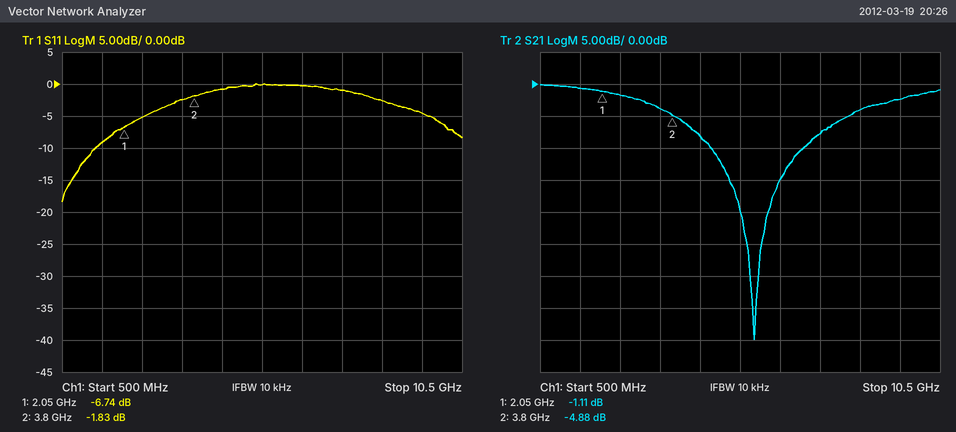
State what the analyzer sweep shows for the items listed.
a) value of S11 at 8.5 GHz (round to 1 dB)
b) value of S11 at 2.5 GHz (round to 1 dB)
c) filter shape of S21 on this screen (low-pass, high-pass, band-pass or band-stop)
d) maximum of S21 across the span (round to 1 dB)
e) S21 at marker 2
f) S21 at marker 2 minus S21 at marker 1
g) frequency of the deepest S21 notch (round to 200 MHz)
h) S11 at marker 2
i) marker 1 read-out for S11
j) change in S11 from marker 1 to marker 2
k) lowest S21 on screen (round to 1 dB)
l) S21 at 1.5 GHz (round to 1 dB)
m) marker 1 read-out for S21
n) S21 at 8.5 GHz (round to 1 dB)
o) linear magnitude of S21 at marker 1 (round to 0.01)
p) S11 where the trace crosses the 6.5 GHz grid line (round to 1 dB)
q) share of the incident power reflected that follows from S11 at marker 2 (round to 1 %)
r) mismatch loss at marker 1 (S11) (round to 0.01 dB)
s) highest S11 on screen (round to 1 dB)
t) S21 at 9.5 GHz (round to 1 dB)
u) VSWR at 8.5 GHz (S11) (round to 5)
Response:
-3 dB
-5 dB
band-stop
0 dB
-4.88 dB
-3.77 dB
5.8 GHz
-1.83 dB
-6.74 dB
4.91 dB
-40 dB
-1 dB
-1.11 dB
-4 dB
0.88
0 dB
66 %
1.03 dB
0 dB
-2 dB
5
